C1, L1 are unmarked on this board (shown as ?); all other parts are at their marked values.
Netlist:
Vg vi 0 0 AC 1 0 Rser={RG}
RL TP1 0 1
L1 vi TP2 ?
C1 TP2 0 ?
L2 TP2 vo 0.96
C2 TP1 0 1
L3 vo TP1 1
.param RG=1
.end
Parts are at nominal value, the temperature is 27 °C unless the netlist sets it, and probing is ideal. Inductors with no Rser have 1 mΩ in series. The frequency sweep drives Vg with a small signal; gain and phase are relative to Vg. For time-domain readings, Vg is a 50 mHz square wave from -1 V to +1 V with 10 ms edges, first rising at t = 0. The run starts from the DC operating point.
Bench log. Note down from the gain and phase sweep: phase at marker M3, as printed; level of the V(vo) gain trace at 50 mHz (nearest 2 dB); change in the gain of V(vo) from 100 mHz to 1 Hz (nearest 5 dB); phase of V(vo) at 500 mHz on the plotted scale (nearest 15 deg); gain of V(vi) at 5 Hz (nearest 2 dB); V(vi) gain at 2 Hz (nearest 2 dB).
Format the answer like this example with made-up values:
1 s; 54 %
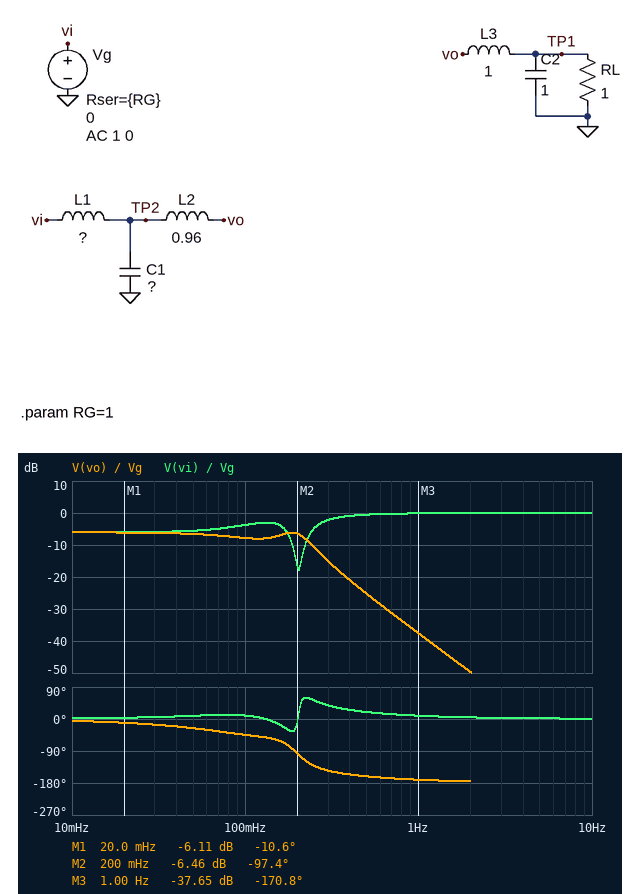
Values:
-170.8 deg; -6 dB; -30 dB; -165 deg; 0 dB; 0 dB
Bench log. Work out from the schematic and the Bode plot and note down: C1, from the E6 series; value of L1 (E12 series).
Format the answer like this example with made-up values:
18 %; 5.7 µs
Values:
1 F; 1 H
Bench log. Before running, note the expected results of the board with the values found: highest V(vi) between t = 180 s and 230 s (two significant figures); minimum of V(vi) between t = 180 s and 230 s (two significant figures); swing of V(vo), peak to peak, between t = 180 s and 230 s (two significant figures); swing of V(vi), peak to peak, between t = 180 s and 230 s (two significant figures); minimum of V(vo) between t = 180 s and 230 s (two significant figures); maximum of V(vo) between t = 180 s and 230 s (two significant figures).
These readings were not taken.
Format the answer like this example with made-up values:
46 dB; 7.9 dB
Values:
1.5 V; -1.5 V; 1.1 V; 3.0 V; -540 mV; 540 mV
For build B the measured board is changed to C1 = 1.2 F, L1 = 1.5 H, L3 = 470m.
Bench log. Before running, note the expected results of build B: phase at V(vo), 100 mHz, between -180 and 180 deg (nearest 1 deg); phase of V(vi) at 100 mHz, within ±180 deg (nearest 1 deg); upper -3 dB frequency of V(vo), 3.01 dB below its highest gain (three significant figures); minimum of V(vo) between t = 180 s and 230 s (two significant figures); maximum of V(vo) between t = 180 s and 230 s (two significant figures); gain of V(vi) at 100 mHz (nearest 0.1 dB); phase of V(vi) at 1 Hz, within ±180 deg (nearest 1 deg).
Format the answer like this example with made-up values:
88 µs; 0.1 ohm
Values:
-74 deg; 17 deg; 139 mHz; -520 mV; 520 mV; -4.5 dB; 6 deg
